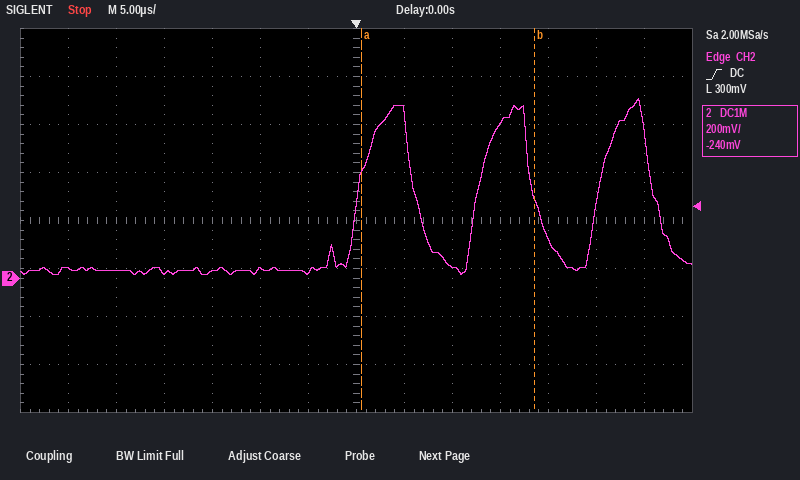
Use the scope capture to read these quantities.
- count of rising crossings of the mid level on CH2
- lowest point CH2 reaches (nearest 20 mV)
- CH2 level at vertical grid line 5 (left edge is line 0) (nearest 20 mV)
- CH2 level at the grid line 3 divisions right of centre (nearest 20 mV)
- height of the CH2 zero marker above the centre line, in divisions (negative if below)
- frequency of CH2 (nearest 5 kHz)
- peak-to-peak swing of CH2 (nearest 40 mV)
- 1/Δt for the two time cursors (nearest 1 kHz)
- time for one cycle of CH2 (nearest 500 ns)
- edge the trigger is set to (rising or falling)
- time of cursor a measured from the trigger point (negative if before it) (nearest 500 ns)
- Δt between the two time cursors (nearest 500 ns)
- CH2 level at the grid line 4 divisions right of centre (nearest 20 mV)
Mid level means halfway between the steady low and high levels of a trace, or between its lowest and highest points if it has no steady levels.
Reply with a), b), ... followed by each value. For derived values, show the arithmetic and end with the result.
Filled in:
a) 3
b) 20 mV
c) 40 mV
d) 640 mV
e) -1.2 div
f) 1 / 12.5 µs ≈ 80 kHz
g) 720 mV
h) 1 / 18.0 µs ≈ 56 kHz
i) 12.5 µs
j) rising
k) +500 ns
l) 18.0 µs
m) 160 mV
